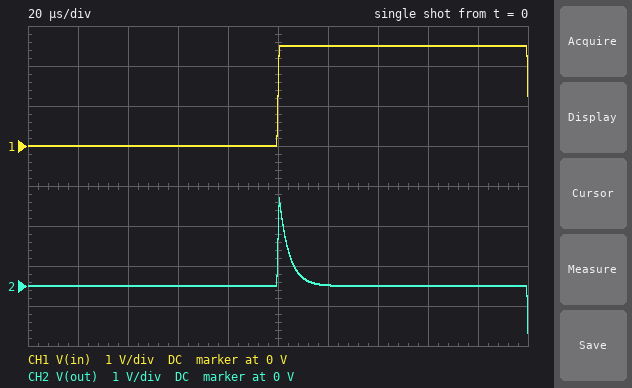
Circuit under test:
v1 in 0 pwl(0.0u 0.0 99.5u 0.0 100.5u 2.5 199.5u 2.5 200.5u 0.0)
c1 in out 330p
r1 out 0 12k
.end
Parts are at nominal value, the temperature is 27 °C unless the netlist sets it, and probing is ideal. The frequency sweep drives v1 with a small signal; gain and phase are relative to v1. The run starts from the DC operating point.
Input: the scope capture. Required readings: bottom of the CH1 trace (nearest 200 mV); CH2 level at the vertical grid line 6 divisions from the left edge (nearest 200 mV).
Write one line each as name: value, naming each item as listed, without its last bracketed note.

bottom of the CH1 trace: 0 V
CH2 level at the vertical grid line 6 divisions from the left edge: 0 V
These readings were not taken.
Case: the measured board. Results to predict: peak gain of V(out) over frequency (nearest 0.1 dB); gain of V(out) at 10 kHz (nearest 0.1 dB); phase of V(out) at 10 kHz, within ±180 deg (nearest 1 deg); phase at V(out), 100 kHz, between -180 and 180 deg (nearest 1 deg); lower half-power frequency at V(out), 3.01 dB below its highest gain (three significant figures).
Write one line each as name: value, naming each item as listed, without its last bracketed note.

peak gain of V(out) over frequency: 0 dB
gain of V(out) at 10 kHz: -12.3 dB
phase of V(out) at 10 kHz, within ±180 deg: 76 deg
phase at V(out), 100 kHz, between -180 and 180 deg: 22 deg
lower half-power frequency at V(out), 3.01 dB below its highest gain: 40.2 kHz
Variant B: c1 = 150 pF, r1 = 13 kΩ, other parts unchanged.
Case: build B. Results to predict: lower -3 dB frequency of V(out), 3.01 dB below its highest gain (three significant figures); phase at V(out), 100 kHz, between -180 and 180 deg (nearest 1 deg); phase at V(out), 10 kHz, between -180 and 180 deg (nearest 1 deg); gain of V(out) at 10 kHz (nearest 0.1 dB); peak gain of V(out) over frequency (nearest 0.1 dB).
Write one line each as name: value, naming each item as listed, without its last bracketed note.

lower -3 dB frequency of V(out), 3.01 dB below its highest gain: 81.6 kHz
phase at V(out), 100 kHz, between -180 and 180 deg: 39 deg
phase at V(out), 10 kHz, between -180 and 180 deg: 83 deg
gain of V(out) at 10 kHz: -18.3 dB
peak gain of V(out) over frequency: 0 dB
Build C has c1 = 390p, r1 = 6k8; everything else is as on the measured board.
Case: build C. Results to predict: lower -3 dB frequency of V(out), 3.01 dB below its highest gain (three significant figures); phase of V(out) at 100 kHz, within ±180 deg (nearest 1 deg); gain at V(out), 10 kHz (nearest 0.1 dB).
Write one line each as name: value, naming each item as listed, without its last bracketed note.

lower -3 dB frequency of V(out), 3.01 dB below its highest gain: 60.0 kHz
phase of V(out) at 100 kHz, within ±180 deg: 31 deg
gain at V(out), 10 kHz: -15.7 dB
